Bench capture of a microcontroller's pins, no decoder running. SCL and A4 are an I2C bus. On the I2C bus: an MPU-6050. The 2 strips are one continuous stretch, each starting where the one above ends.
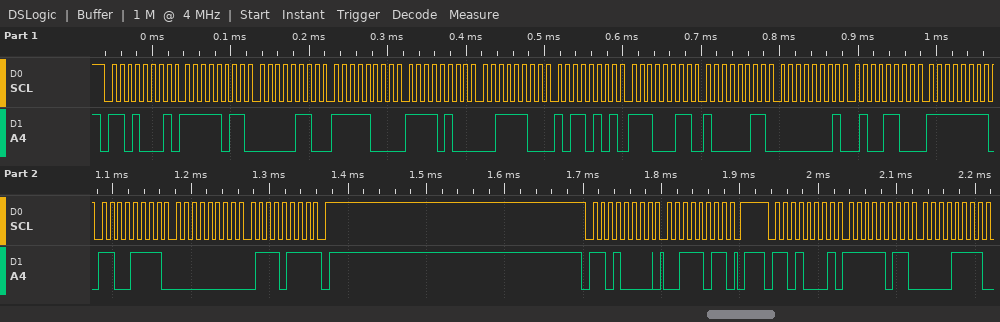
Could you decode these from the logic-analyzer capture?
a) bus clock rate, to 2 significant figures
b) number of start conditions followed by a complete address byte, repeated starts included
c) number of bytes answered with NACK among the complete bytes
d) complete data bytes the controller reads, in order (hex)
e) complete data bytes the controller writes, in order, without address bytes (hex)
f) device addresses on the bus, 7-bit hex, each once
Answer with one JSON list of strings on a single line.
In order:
["100 kHz", "3", "1", "FB 06 F8 F4 3C B5 E3 83 01 4C FF CF 00 77 FB 0F", "3B", "0x68"]
